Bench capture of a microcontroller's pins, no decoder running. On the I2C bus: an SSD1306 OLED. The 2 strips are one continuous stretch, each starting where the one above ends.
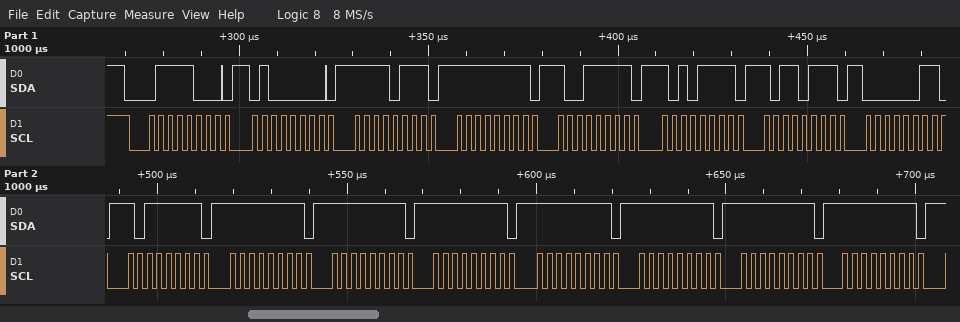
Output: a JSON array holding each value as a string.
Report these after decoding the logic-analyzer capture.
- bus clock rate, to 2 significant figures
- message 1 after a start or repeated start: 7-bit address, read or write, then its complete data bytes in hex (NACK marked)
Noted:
["400 kHz", "0x3C write: 40 F7 FF 9F AF B7 03 BF FF FF FF FF FF FF FF"]
